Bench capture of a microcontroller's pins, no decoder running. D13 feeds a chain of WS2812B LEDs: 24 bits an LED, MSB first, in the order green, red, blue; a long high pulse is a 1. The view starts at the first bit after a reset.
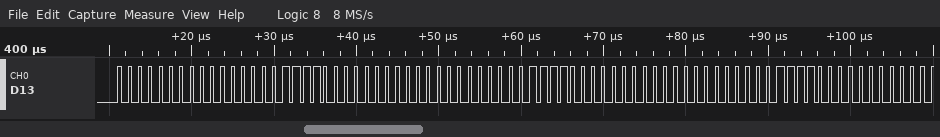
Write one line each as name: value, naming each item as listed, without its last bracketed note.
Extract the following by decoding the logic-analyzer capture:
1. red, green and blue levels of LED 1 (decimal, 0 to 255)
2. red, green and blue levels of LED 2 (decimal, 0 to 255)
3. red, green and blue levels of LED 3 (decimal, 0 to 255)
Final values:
red, green and blue levels of LED 1: 0, 0, 240
red, green and blue levels of LED 2: 0, 0, 240
red, green and blue levels of LED 3: 0, 0, 240
